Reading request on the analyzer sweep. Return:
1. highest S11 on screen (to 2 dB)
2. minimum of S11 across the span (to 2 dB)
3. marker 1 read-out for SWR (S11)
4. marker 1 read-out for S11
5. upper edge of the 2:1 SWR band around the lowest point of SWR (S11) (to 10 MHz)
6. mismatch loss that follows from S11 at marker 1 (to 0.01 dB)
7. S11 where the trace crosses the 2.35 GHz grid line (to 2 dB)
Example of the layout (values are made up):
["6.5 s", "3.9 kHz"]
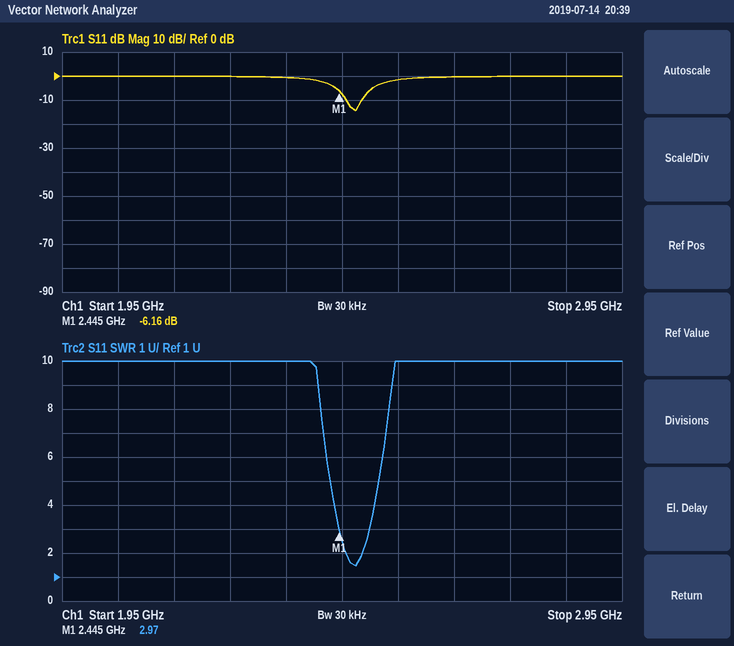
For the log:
["0 dB", "-14 dB", "2.97", "-6.16 dB", "2.49 GHz", "1.20 dB", "0 dB"]
